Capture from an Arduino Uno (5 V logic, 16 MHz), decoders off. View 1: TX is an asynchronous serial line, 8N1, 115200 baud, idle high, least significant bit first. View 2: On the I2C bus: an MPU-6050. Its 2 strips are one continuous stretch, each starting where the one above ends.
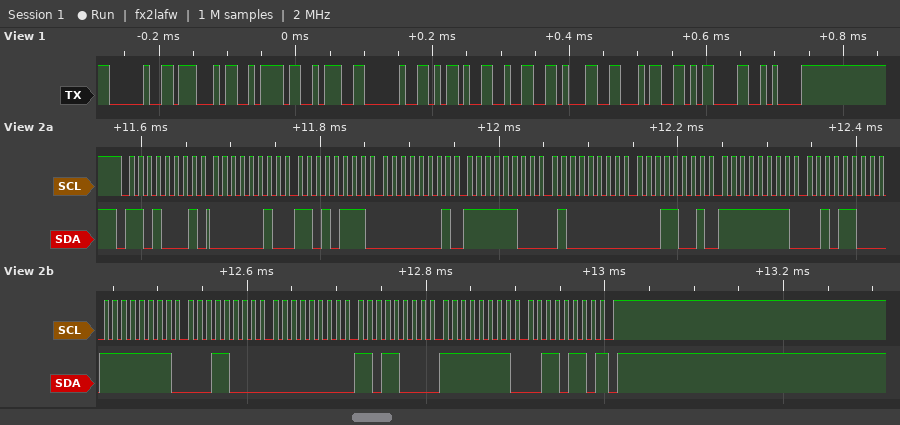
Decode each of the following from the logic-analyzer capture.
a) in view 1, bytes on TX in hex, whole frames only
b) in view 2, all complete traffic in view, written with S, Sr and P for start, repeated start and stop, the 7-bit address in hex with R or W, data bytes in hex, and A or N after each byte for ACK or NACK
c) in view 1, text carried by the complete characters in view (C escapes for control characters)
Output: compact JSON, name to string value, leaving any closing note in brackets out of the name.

{"in view 1, bytes on TX in hex, whole frames only": "20 47 7A 3A 20 2D 32 31 34 0D 0A", "in view 2, all complete traffic in view, written with S, Sr and P for start, repeated start and stop, the 7-bit address in hex with R or W, data bytes in hex, and A or N after each byte for ACK or NACK": "S 68R A 02 A D7 A 01 A FC A 40 A 19 A FF A 2C A FF A 18 A 00 A D8 A FF A 36 N P", "in view 1, text carried by the complete characters in view": "\" Gz: -214\\r\\n\""}
